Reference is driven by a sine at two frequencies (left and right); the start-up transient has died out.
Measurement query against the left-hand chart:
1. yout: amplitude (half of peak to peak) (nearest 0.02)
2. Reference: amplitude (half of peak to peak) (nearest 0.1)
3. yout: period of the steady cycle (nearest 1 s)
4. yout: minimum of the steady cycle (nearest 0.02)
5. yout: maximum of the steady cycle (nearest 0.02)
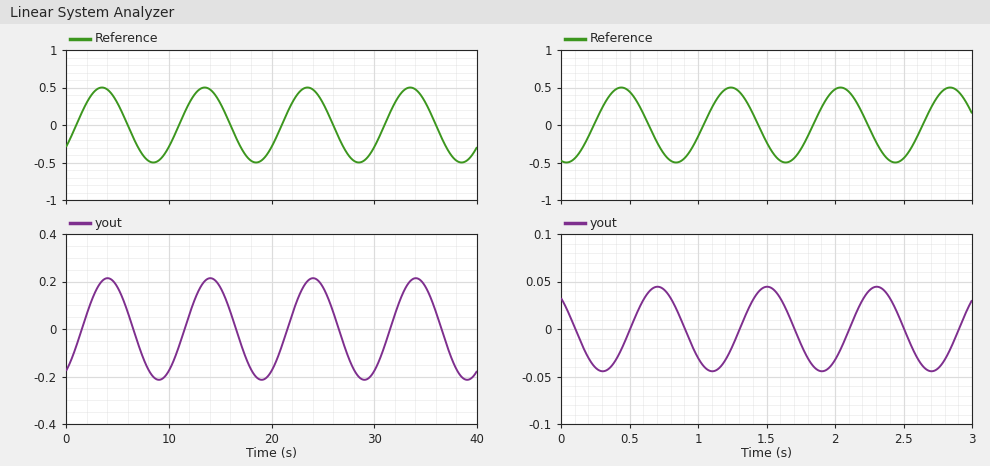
0.22
0.5
10 s
-0.22
0.22
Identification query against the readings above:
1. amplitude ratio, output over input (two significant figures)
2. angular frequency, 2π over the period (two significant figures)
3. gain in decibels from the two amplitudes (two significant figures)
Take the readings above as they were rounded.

0.44
0.63 rad/s
-7.1 dB
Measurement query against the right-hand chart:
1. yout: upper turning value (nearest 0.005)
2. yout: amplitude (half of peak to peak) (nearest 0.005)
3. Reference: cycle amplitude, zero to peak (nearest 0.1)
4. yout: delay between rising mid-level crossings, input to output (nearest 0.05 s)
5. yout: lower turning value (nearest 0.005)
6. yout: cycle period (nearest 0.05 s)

0.045
0.045
0.5
0.25 s
-0.045
0.80 s
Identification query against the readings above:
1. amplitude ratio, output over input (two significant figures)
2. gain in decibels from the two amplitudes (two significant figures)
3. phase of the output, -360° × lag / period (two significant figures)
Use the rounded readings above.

0.090
-21 dB
-110°
